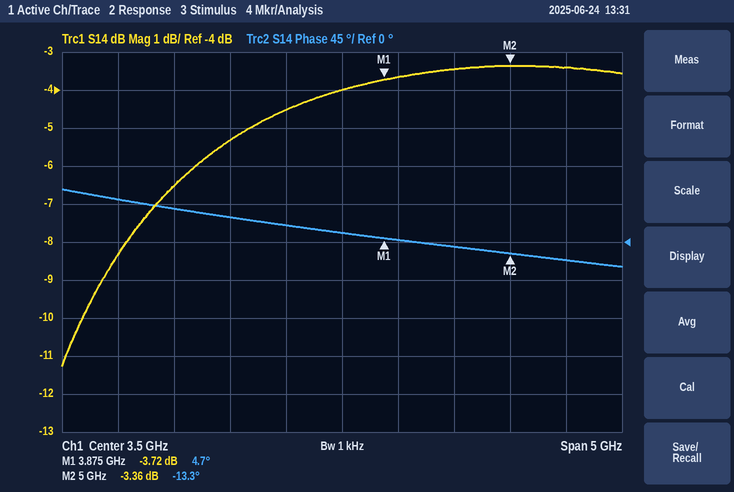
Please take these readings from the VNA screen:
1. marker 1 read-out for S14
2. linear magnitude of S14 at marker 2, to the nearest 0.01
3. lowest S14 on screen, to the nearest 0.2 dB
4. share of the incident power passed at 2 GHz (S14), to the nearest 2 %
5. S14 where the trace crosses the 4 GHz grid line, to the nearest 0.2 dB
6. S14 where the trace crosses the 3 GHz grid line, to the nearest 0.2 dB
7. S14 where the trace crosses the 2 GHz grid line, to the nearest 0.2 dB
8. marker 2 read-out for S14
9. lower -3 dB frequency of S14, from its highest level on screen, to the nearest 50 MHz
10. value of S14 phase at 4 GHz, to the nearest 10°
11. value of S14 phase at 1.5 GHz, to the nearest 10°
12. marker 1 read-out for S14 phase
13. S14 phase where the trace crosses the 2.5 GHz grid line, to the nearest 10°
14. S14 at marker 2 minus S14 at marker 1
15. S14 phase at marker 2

-3.72 dB
0.68
-11.2 dB
22 %
-3.6 dB
-4.6 dB
-6.6 dB
-3.36 dB
2.05 GHz
0°
50°
4.7°
30°
0.36 dB
-13.3°
